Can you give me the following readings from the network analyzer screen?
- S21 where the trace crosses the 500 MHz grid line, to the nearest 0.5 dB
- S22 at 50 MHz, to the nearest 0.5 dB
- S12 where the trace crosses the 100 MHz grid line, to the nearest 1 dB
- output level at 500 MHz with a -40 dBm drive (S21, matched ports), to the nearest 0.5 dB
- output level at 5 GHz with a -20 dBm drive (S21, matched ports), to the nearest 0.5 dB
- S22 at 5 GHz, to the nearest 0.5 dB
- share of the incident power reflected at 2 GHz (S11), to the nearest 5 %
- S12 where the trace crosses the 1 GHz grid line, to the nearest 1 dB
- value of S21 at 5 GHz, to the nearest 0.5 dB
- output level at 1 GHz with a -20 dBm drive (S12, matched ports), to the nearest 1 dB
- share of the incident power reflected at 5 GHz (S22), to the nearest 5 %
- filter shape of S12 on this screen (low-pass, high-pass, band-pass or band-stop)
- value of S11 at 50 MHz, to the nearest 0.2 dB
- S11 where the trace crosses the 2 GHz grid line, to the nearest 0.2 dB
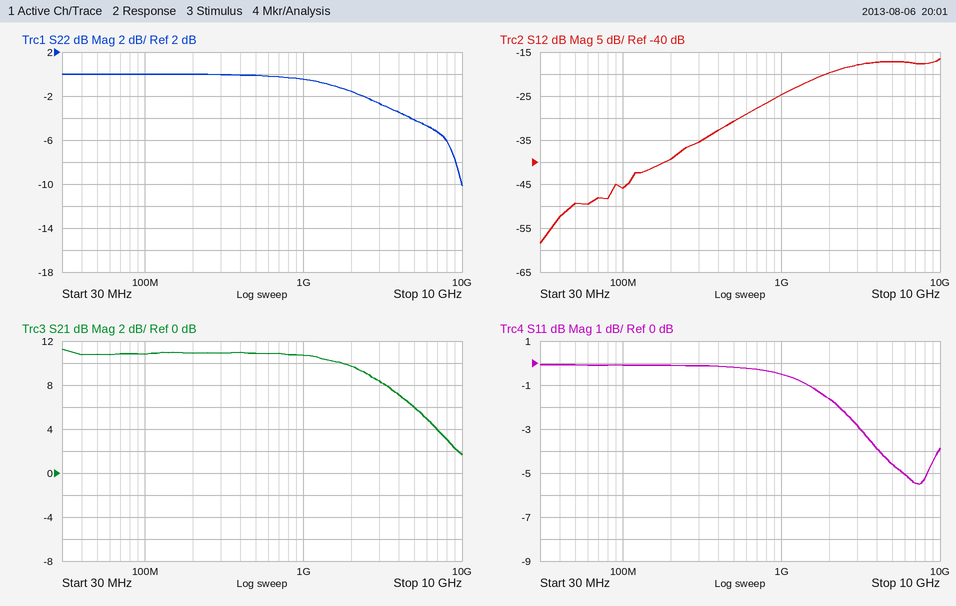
11.0 dB
0.0 dB
-46 dB
-29.0 dBm
-14.0 dBm
-4.0 dB
70 %
-25 dB
6.0 dB
-45 dBm
40 %
high-pass
0.0 dB
-1.6 dB
